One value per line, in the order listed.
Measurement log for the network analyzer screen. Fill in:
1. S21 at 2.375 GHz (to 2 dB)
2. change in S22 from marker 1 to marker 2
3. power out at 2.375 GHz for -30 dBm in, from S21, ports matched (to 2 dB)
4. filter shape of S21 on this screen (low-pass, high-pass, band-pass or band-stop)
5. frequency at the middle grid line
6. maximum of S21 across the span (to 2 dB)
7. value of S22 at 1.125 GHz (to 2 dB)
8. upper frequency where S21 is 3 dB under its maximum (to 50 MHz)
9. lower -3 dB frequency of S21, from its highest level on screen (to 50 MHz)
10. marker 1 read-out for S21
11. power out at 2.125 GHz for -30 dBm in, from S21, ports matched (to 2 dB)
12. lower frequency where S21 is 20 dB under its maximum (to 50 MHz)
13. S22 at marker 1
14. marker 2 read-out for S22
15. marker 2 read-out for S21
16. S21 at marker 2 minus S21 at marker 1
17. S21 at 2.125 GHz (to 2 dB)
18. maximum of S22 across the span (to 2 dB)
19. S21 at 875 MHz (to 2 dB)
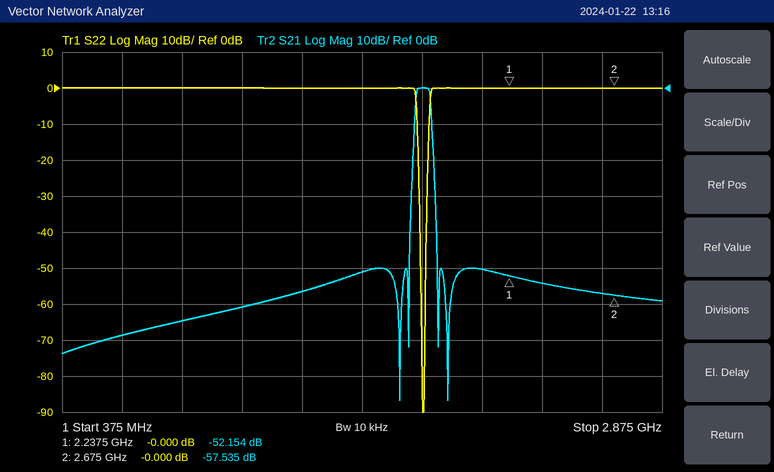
-54 dB
0.000 dB
-84 dBm
band-pass
1.625 GHz
0 dB
0 dB
1.90 GHz
1.85 GHz
-52.154 dB
-80 dBm
1.85 GHz
-0.000 dB
-0.000 dB
-57.535 dB
-5.381 dB
-50 dB
0 dB
-64 dB
